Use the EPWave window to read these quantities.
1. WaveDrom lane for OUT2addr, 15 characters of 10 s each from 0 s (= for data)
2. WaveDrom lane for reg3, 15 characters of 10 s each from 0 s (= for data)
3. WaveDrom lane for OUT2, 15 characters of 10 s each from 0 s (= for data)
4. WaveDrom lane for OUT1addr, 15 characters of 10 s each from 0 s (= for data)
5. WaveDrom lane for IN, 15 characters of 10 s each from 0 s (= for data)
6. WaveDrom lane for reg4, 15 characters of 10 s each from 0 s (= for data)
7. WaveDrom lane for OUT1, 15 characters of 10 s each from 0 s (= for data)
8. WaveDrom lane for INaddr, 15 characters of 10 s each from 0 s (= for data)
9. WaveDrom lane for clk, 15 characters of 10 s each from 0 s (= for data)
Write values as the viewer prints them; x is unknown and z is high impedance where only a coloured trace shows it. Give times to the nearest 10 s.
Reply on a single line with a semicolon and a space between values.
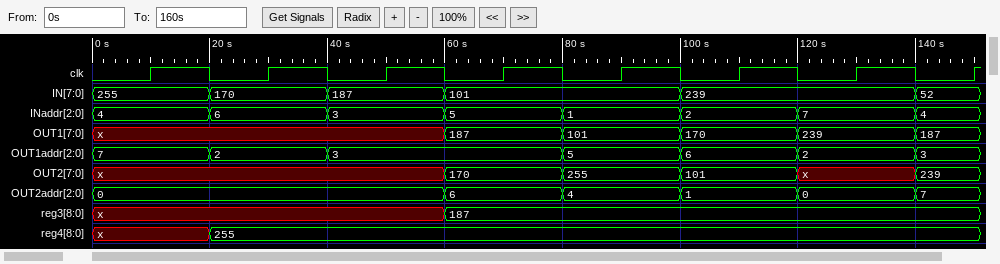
{name: 'OUT2addr', wave: '=.....=.=.=.=.=', data: '0 6 4 1 0 7'}; {name: 'reg3', wave: 'x.....=........', data: '187'}; {name: 'OUT2', wave: 'x.....=.=.=.x.=', data: '170 255 101 239'}; {name: 'OUT1addr', wave: '=.=.=...=.=.=.=', data: '7 2 3 5 6 2 3'}; {name: 'IN', wave: '=.=.=.=...=...=', data: '255 170 187 101 239 52'}; {name: 'reg4', wave: 'x.=............', data: '255'}; {name: 'OUT1', wave: 'x.....=.=.=.=.=', data: '187 101 170 239 187'}; {name: 'INaddr', wave: '=.=.=.=.=.=.=.=', data: '4 6 3 5 1 2 7 4'}; {name: 'clk', wave: '010101010101010'}
